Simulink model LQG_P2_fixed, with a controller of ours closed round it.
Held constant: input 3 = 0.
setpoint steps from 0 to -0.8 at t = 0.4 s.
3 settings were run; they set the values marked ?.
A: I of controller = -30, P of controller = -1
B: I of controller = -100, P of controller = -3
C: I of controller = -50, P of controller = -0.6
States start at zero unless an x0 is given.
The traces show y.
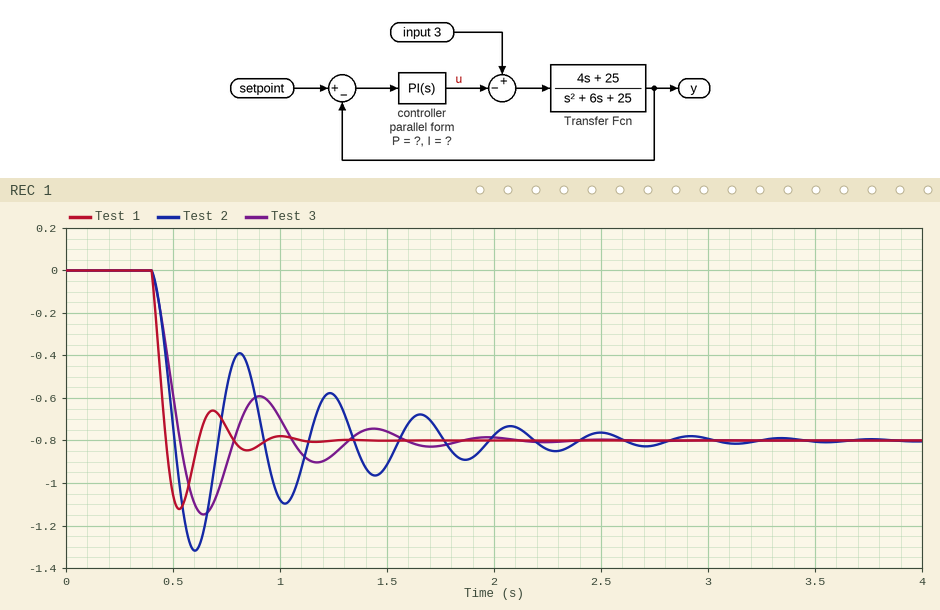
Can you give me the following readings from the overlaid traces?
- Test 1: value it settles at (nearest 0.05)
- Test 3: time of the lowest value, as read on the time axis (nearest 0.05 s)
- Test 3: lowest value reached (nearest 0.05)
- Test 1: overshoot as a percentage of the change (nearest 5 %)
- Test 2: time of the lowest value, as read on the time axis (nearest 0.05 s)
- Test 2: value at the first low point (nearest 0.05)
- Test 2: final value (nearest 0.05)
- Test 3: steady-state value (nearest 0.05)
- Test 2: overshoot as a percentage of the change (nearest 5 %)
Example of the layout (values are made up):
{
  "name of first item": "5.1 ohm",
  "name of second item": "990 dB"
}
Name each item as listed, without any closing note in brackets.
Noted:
{
  "Test 1: value it settles at": "-0.80",
  "Test 3: time of the lowest value, as read on the time axis": "0.65 s",
  "Test 3: lowest value reached": "-1.15",
  "Test 1: overshoot as a percentage of the change": "40 %",
  "Test 2: time of the lowest value, as read on the time axis": "0.60 s",
  "Test 2: value at the first low point": "-1.30",
  "Test 2: final value": "-0.80",
  "Test 3: steady-state value": "-0.80",
  "Test 2: overshoot as a percentage of the change": "65 %"
}
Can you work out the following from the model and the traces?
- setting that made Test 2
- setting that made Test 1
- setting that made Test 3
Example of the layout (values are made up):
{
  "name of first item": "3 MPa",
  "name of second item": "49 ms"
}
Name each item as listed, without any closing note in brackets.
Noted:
{
  "setting that made Test 2": "C",
  "setting that made Test 1": "B",
  "setting that made Test 3": "A"
}
